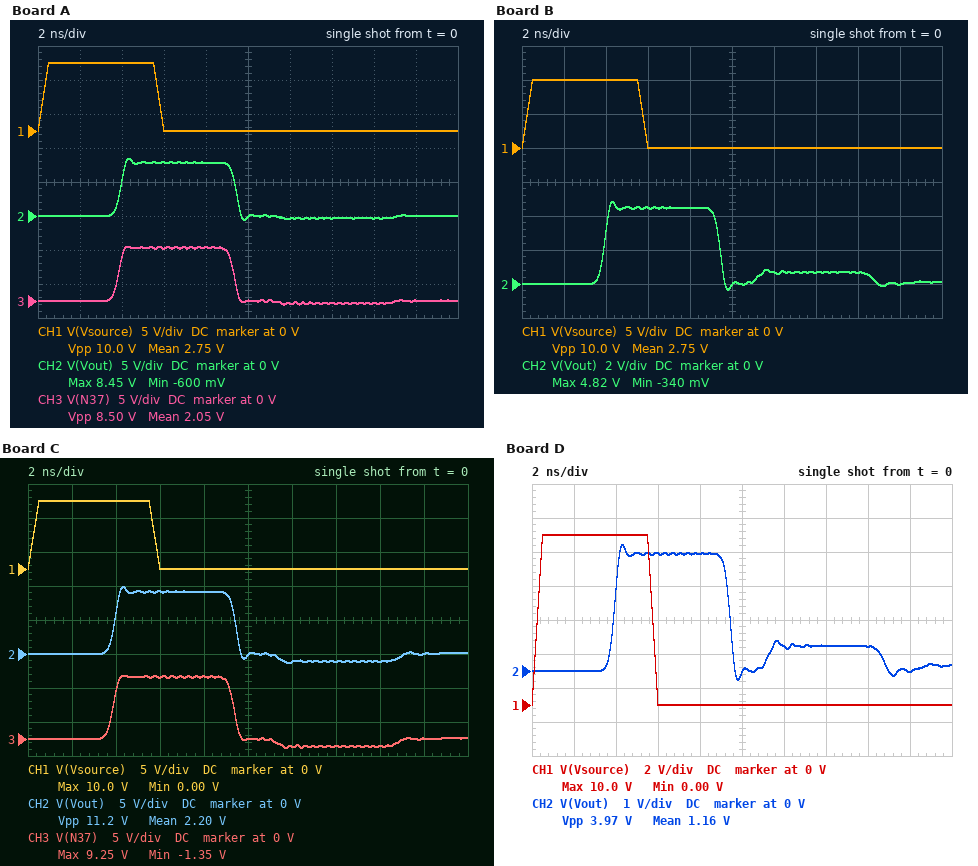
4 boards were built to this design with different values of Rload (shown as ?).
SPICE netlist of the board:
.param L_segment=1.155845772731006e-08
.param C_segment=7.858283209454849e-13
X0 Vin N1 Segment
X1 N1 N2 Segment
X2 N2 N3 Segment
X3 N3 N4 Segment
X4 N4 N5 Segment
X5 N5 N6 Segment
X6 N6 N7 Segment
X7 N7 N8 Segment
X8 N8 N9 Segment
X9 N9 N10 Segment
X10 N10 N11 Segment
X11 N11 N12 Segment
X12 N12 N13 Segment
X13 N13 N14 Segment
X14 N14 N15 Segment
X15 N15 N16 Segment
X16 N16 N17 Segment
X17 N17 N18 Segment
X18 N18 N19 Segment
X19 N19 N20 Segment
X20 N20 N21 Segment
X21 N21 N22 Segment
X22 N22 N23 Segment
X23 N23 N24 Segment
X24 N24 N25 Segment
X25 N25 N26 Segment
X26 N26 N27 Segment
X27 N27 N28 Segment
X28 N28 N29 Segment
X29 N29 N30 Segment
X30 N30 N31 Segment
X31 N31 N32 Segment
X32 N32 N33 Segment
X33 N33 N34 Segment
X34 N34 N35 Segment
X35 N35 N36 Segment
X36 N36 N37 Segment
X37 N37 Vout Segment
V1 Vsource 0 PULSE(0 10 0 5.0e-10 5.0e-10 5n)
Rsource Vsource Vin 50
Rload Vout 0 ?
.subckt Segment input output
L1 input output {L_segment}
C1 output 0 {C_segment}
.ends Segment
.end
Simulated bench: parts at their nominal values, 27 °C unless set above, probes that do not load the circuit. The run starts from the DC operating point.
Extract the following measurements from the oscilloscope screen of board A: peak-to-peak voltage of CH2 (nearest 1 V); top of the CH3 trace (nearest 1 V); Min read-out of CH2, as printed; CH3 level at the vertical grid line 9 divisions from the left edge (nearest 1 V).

9 V
8 V
-600 mV
0 V
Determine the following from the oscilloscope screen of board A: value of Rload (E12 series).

150 Ω
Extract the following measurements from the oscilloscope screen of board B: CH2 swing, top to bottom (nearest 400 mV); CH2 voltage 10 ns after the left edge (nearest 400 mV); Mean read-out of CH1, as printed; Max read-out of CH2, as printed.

5.2 V
0 V
2.75 V
4.82 V
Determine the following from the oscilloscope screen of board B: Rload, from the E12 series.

56 Ω
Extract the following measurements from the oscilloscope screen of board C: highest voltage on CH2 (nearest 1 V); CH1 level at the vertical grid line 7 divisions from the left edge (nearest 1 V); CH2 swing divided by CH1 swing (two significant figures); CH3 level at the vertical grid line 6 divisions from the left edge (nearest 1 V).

10 V
0 V
1.1
-1 V
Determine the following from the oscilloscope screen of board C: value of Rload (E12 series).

220 Ω
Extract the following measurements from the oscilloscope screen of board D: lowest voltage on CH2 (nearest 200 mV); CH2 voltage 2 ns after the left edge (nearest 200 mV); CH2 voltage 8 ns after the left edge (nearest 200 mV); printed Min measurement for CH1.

-200 mV
0 V
3.4 V
0.00 V
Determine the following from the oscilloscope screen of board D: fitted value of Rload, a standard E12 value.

39 Ω
